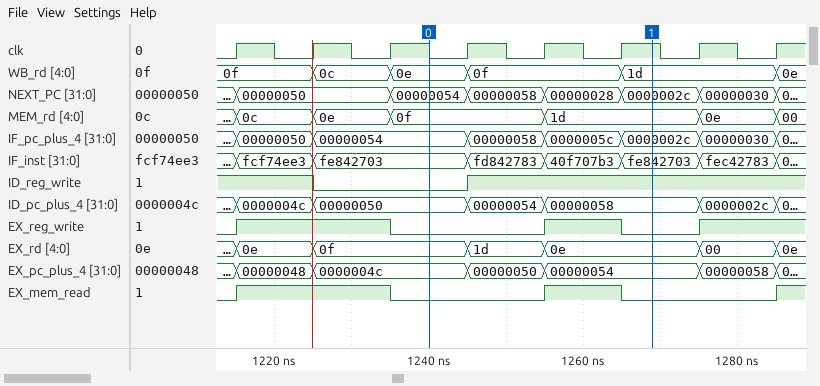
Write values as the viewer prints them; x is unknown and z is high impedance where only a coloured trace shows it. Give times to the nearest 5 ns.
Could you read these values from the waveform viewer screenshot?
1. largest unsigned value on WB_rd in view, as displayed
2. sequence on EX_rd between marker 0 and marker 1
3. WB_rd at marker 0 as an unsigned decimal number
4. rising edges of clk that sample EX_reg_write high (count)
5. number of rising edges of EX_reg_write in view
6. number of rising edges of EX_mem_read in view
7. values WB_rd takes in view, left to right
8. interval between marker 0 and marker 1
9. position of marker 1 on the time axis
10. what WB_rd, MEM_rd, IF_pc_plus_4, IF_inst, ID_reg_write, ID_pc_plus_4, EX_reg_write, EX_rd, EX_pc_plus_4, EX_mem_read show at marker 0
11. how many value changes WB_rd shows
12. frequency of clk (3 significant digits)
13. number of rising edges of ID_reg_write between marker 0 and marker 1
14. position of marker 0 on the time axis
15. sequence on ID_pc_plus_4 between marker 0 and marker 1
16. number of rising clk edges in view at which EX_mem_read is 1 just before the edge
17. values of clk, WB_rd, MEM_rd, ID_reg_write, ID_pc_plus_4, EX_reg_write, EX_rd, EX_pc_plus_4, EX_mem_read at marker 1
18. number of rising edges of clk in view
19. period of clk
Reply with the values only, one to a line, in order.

1d
0f, 1d, 0e
14
4
3
3
0f, 0c, 0e, 0f, 1d, 0e
30 ns
1270 ns
WB_rd=0e, MEM_rd=0f, IF_pc_plus_4=00000054, IF_inst=fe842703, ID_reg_write=0, ID_pc_plus_4=00000050, EX_reg_write=0, EX_rd=0f, EX_pc_plus_4=0000004c, EX_mem_read=0
5
100 MHz
1
1240 ns
00000050, 00000054, 00000058
3
clk=1, WB_rd=1d, MEM_rd=1d, ID_reg_write=1, ID_pc_plus_4=00000058, EX_reg_write=0, EX_rd=0e, EX_pc_plus_4=00000054, EX_mem_read=0
8
10 ns
